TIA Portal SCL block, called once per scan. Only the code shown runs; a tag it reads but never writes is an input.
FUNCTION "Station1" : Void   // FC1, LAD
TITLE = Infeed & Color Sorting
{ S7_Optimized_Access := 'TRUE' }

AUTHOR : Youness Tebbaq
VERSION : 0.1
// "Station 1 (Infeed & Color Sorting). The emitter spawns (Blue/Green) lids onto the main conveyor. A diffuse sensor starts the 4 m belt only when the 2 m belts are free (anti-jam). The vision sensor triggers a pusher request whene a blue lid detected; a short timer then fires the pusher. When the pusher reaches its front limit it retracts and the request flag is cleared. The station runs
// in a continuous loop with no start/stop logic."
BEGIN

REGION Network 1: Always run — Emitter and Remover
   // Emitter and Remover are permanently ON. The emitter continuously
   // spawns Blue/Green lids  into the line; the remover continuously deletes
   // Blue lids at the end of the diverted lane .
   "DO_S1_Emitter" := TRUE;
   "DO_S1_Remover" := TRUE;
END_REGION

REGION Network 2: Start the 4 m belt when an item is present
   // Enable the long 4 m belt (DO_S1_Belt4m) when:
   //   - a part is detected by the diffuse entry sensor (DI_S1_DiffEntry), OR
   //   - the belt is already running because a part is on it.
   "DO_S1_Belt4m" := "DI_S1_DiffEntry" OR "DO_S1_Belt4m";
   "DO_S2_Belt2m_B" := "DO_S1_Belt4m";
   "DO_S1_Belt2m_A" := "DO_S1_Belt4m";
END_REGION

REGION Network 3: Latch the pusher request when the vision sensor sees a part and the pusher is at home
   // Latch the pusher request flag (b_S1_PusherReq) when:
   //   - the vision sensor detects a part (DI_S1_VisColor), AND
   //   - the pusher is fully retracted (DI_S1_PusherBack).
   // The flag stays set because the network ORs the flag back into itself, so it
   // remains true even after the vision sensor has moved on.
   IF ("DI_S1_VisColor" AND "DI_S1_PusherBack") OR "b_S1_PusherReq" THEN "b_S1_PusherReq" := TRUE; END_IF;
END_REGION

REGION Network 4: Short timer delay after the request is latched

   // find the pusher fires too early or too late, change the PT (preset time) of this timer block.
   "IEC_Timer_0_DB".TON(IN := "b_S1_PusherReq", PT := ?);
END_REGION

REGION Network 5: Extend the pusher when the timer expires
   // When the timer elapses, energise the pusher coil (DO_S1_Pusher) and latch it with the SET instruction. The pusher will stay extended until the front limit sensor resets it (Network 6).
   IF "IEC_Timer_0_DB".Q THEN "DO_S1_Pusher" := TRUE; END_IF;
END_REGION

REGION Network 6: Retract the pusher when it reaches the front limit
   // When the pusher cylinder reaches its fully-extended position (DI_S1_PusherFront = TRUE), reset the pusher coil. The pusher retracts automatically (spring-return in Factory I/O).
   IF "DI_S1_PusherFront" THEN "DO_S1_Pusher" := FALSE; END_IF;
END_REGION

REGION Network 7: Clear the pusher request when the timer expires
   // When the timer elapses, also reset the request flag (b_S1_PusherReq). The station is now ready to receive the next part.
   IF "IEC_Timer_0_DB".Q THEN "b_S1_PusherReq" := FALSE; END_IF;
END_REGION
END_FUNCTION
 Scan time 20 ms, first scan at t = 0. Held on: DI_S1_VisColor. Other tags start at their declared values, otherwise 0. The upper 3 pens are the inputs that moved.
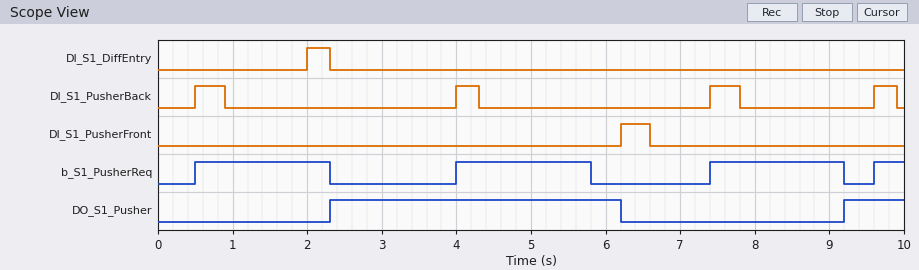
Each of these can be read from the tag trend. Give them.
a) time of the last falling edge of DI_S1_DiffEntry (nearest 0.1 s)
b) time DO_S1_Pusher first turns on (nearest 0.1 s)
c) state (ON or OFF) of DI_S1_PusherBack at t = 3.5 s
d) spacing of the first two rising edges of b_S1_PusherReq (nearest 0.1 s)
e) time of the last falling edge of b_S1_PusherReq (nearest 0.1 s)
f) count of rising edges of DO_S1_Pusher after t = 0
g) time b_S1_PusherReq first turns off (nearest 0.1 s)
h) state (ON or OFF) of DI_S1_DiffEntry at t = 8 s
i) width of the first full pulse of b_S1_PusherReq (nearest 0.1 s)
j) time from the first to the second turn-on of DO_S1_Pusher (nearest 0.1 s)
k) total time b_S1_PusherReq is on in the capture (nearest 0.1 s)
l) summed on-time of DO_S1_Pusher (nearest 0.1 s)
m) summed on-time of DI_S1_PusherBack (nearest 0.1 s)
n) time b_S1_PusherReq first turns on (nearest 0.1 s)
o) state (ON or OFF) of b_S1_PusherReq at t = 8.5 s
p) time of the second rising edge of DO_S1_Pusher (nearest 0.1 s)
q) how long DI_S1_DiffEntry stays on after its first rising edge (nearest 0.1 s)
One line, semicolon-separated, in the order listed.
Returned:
2.3 s; 2.3 s; OFF; 3.5 s; 9.2 s; 2; 2.3 s; OFF; 1.8 s; 6.9 s; 5.8 s; 4.7 s; 1.4 s; 0.5 s; ON; 9.2 s; 0.3 s
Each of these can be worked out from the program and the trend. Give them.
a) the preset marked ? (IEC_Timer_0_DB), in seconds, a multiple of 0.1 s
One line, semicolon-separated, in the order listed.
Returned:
1.8 s
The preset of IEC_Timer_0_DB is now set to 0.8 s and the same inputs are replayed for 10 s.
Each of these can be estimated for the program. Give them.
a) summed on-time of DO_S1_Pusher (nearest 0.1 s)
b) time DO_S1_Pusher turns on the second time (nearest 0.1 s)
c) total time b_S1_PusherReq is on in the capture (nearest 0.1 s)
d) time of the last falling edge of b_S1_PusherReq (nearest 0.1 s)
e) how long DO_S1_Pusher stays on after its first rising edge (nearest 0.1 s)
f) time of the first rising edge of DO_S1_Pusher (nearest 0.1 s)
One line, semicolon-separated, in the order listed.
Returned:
6.7 s; 8.2 s; 2.8 s; 8.2 s; 4.9 s; 1.3 s
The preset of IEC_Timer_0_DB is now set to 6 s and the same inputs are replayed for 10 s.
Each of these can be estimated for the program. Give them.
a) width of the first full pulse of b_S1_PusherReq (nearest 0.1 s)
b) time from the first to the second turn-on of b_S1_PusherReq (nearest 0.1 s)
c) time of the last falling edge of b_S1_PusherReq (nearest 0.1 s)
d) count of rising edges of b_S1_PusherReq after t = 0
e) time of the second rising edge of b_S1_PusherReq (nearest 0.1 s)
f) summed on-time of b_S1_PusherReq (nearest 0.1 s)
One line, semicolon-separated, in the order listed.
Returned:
6.0 s; 6.9 s; 6.5 s; 2; 7.4 s; 8.6 s
